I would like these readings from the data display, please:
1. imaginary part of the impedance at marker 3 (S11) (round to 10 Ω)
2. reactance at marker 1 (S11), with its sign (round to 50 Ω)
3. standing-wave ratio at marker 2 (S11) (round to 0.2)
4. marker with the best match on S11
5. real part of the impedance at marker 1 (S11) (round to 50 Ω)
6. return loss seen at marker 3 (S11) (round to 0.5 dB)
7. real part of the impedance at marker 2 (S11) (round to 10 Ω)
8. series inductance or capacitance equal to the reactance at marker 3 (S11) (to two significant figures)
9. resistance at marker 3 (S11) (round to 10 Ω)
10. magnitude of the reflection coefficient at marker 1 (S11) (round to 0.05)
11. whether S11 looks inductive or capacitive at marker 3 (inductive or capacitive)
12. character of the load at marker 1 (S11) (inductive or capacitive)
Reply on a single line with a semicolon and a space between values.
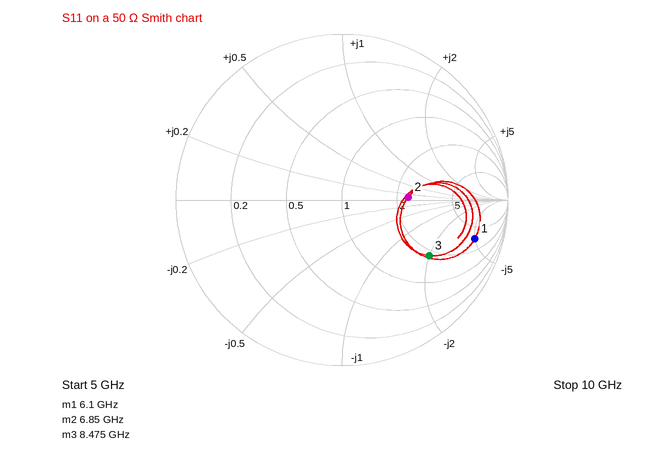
-100 Ω; -250 Ω; 2.4; marker 2; 150 Ω; 4.0 dB; 120 Ω; 190 fF; 90 Ω; 0.85; capacitive; capacitive
